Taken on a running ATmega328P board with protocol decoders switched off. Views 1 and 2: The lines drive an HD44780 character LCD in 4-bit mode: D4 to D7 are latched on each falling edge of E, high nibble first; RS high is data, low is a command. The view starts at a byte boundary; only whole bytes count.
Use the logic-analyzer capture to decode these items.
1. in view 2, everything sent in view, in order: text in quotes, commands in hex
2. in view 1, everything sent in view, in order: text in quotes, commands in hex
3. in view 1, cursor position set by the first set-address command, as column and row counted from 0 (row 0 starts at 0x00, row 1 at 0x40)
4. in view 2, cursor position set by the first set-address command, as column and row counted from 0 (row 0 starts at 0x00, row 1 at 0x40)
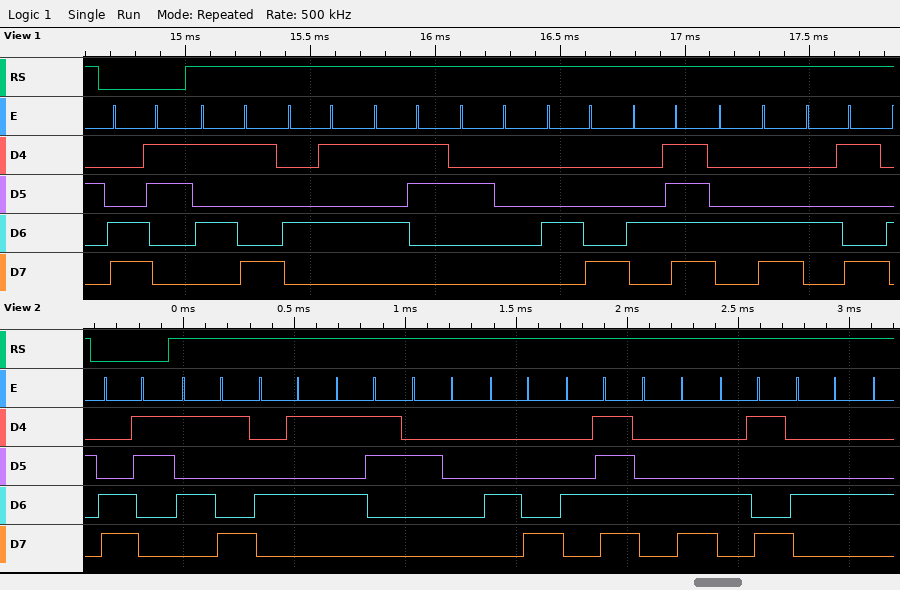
0xC3 "YES HOLID"
0xC3 "YES HOLI"
column 3, row 1
column 3, row 1
